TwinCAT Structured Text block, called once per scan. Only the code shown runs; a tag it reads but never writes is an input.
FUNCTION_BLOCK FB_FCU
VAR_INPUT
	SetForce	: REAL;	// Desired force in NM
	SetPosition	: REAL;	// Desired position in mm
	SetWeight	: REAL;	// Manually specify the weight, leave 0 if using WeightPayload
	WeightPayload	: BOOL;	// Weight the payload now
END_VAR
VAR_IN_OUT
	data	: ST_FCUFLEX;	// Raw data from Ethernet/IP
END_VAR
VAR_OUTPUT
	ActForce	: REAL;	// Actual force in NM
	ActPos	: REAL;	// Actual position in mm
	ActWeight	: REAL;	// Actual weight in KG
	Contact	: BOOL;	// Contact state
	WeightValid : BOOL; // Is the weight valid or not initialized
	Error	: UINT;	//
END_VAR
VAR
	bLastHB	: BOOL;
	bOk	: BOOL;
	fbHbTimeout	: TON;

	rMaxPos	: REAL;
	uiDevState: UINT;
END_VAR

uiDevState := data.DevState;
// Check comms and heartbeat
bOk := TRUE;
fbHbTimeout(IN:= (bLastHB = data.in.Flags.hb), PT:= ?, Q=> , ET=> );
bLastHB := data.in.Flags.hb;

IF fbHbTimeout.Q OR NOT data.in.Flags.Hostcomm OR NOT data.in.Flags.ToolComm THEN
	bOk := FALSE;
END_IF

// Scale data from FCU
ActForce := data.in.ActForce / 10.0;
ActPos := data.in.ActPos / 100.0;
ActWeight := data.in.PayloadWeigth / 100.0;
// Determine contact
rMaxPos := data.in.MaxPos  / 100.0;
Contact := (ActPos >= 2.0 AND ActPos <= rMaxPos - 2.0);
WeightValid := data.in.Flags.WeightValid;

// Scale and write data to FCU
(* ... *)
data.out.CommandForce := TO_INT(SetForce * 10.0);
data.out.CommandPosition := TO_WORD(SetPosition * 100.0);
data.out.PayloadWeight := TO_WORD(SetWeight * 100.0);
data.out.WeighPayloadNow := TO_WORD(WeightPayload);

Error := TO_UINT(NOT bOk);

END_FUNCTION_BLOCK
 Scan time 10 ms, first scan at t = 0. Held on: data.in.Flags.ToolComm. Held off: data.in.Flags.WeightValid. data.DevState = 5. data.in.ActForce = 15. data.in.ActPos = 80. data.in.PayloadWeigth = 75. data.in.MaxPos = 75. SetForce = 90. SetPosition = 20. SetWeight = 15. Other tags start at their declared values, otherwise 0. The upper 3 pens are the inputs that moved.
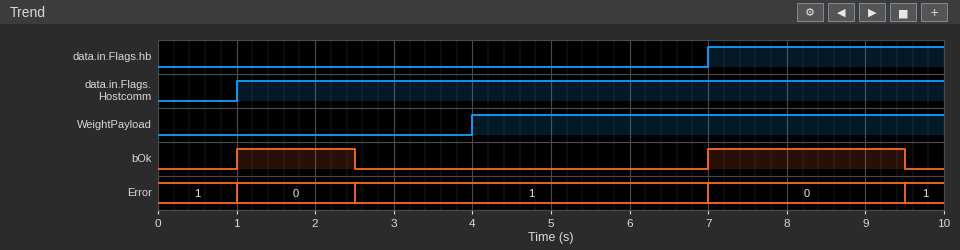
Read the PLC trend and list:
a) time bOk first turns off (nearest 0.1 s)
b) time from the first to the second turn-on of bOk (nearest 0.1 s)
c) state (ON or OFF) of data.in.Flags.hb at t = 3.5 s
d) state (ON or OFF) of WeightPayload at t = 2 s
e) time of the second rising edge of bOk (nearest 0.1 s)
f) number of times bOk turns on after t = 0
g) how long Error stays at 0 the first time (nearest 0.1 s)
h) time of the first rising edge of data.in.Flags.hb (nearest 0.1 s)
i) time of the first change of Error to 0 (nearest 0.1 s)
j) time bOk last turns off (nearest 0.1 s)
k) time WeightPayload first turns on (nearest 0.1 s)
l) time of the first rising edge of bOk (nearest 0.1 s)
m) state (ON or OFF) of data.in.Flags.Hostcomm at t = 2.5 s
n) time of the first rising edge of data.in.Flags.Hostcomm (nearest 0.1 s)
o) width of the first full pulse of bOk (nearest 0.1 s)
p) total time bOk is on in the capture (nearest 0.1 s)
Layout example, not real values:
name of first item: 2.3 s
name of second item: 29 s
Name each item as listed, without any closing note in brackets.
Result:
time bOk first turns off: 2.5 s
time from the first to the second turn-on of bOk: 6.0 s
state (ON or OFF) of data.in.Flags.hb at t = 3.5 s: OFF
state (ON or OFF) of WeightPayload at t = 2 s: OFF
time of the second rising edge of bOk: 7.0 s
number of times bOk turns on after t = 0: 2
how long Error stays at 0 the first time: 1.5 s
time of the first rising edge of data.in.Flags.hb: 7.0 s
time of the first change of Error to 0: 1.0 s
time bOk last turns off: 9.5 s
time WeightPayload first turns on: 4.0 s
time of the first rising edge of bOk: 1.0 s
state (ON or OFF) of data.in.Flags.Hostcomm at t = 2.5 s: ON
time of the first rising edge of data.in.Flags.Hostcomm: 1.0 s
width of the first full pulse of bOk: 1.5 s
total time bOk is on in the capture: 4.0 s
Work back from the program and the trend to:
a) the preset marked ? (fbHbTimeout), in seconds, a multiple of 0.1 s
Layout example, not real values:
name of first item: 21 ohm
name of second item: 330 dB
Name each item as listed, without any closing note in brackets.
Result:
the preset marked ? (fbHbTimeout), in seconds, a multiple of 0.1 s: 2.5 s
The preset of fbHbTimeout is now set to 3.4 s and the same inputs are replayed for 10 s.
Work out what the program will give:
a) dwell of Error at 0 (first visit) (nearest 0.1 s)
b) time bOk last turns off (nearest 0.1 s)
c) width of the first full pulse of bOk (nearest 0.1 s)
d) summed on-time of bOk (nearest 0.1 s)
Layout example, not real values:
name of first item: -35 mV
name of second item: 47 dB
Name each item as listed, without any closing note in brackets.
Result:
dwell of Error at 0 (first visit): 2.4 s
time bOk last turns off: 3.4 s
width of the first full pulse of bOk: 2.4 s
summed on-time of bOk: 5.4 s
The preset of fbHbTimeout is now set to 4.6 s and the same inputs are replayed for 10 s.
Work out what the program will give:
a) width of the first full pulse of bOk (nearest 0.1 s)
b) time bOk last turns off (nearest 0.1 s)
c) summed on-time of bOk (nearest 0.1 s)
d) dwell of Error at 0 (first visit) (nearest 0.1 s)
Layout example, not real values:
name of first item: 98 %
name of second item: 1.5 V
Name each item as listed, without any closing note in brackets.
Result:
width of the first full pulse of bOk: 3.6 s
time bOk last turns off: 4.6 s
summed on-time of bOk: 6.6 s
dwell of Error at 0 (first visit): 3.6 s
